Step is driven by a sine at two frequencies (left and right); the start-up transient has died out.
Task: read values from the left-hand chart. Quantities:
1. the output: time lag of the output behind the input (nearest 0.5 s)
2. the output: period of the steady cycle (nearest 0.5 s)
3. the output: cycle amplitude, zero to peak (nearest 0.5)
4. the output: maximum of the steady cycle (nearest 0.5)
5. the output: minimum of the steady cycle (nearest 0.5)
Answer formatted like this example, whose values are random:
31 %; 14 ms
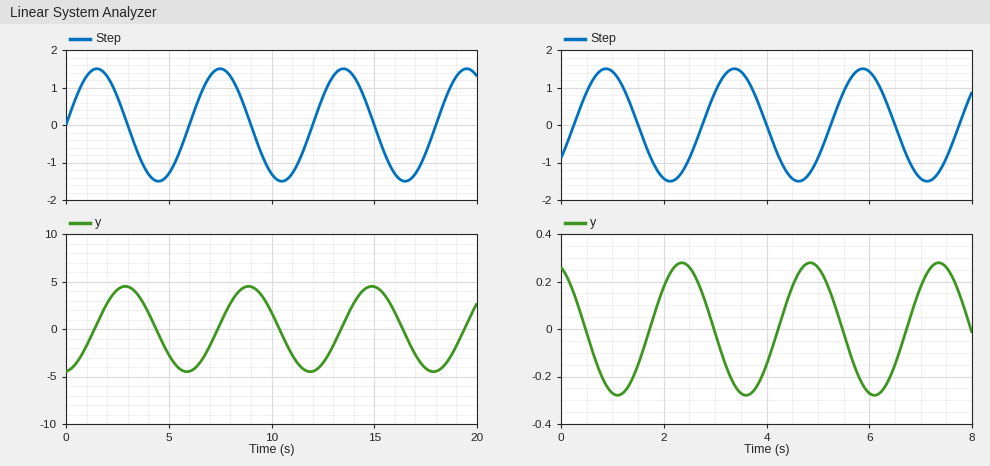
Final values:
1.5 s; 6.0 s; 4.5; 4.5; -4.5
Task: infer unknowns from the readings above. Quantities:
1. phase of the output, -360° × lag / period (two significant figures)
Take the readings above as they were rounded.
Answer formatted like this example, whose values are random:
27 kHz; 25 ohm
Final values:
-90°
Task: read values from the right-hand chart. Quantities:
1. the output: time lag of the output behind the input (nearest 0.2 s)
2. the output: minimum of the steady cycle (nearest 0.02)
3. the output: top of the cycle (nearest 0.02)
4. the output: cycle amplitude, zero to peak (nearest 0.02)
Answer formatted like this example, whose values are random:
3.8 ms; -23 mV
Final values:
1.4 s; -0.28; 0.28; 0.28
